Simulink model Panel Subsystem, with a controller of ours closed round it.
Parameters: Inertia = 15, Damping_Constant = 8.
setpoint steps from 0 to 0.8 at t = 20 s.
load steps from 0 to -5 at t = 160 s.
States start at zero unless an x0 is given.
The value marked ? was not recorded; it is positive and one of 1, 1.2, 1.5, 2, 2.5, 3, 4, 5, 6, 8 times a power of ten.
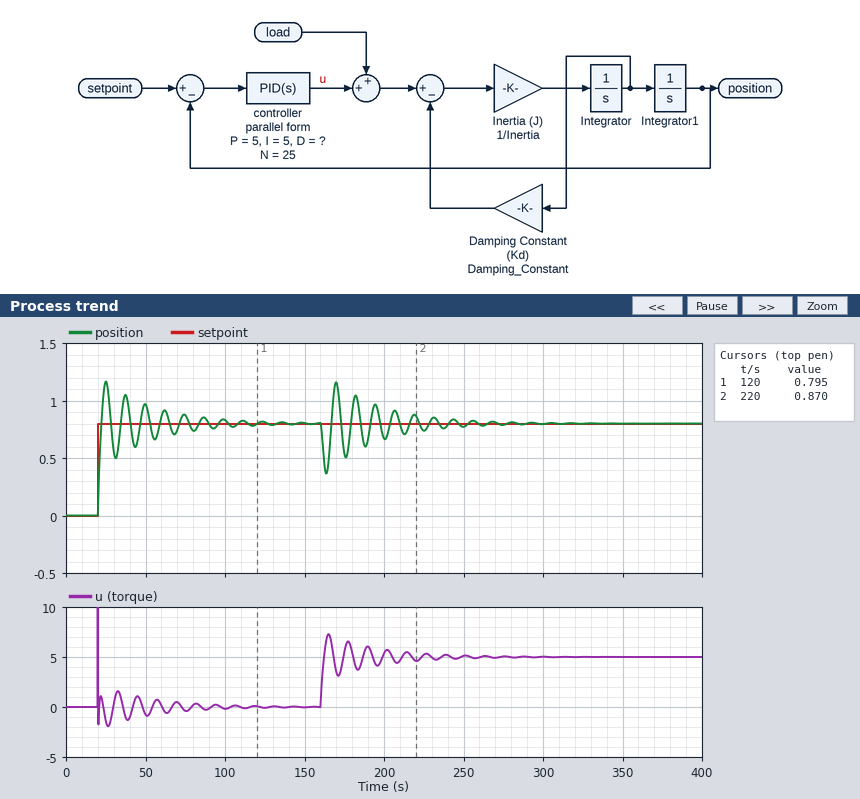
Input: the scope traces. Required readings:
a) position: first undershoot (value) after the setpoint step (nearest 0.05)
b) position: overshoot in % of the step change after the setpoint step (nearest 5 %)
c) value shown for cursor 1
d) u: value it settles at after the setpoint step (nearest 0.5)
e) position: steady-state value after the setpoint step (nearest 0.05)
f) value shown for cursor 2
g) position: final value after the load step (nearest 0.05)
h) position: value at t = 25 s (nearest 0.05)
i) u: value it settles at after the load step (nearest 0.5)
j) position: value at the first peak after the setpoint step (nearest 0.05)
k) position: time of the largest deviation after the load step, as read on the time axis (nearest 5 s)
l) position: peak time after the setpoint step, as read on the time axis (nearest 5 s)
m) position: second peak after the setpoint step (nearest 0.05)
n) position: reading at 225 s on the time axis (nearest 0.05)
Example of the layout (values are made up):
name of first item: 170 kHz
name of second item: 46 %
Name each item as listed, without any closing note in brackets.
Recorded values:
position: first undershoot (value) after the setpoint step: 0.50
position: overshoot in % of the step change after the setpoint step: 45 %
value shown for cursor 1: 0.795
u: value it settles at after the setpoint step: 0.0
position: steady-state value after the setpoint step: 0.80
value shown for cursor 2: 0.870
position: final value after the load step: 0.80
position: value at t = 25 s: 1.15
u: value it settles at after the load step: 5.0
position: value at the first peak after the setpoint step: 1.15
position: time of the largest deviation after the load step, as read on the time axis: 165 s
position: peak time after the setpoint step, as read on the time axis: 25 s
position: second peak after the setpoint step: 1.05
position: reading at 225 s on the time axis: 0.75
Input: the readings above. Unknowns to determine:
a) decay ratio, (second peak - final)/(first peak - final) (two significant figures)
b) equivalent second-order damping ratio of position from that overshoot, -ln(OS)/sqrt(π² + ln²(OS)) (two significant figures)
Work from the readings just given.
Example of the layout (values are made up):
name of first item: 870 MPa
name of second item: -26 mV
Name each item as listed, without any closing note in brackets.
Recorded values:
decay ratio, (second peak - final)/(first peak - final): 0.71
equivalent second-order damping ratio of position from that overshoot, -ln(OS)/sqrt(π² + ln²(OS)): 0.25
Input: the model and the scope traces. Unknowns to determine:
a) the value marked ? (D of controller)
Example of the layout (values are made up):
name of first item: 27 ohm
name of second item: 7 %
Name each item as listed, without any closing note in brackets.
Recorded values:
the value marked ?: 12
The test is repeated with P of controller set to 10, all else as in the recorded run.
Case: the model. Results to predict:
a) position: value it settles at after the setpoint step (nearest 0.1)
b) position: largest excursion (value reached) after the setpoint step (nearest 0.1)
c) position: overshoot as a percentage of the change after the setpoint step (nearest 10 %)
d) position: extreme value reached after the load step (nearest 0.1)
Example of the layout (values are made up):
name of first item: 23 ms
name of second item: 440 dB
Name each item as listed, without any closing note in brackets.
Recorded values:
position: value it settles at after the setpoint step: 0.8
position: largest excursion (value reached) after the setpoint step: 1.1
position: overshoot as a percentage of the change after the setpoint step: 30 %
position: extreme value reached after the load step: 0.5
